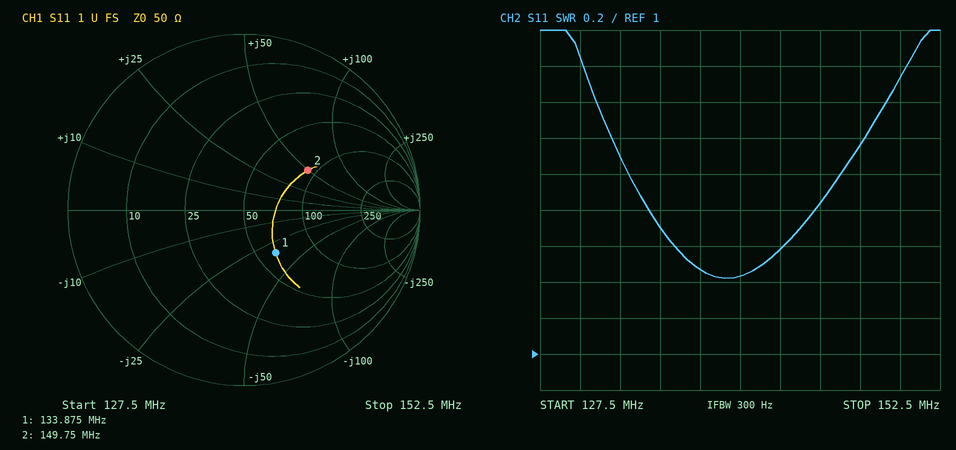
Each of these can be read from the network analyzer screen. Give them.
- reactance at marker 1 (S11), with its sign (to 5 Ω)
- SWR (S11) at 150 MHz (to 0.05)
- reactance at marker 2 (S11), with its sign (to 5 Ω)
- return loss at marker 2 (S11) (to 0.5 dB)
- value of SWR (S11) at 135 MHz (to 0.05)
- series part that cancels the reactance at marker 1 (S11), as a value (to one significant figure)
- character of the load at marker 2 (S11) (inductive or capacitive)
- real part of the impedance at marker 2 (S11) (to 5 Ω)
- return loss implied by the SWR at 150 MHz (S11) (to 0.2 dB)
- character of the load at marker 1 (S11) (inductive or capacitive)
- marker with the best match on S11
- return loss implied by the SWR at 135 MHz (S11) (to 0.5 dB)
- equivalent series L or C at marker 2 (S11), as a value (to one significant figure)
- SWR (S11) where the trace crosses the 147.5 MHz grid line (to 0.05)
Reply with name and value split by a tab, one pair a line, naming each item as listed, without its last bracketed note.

reactance at marker 1 (S11), with its sign	-35 Ω
SWR (S11) at 150 MHz	2.55
reactance at marker 2 (S11), with its sign	+50 Ω
return loss at marker 2 (S11)	7.5 dB
value of SWR (S11) at 135 MHz	1.70
series part that cancels the reactance at marker 1 (S11), as a value	40 nH
character of the load at marker 2 (S11)	inductive
real part of the impedance at marker 2 (S11)	90 Ω
return loss implied by the SWR at 150 MHz (S11)	7.2 dB
character of the load at marker 1 (S11)	capacitive
marker with the best match on S11	marker 1
return loss implied by the SWR at 135 MHz (S11)	11.5 dB
equivalent series L or C at marker 2 (S11), as a value	50 nH
SWR (S11) where the trace crosses the 147.5 MHz grid line	2.15
